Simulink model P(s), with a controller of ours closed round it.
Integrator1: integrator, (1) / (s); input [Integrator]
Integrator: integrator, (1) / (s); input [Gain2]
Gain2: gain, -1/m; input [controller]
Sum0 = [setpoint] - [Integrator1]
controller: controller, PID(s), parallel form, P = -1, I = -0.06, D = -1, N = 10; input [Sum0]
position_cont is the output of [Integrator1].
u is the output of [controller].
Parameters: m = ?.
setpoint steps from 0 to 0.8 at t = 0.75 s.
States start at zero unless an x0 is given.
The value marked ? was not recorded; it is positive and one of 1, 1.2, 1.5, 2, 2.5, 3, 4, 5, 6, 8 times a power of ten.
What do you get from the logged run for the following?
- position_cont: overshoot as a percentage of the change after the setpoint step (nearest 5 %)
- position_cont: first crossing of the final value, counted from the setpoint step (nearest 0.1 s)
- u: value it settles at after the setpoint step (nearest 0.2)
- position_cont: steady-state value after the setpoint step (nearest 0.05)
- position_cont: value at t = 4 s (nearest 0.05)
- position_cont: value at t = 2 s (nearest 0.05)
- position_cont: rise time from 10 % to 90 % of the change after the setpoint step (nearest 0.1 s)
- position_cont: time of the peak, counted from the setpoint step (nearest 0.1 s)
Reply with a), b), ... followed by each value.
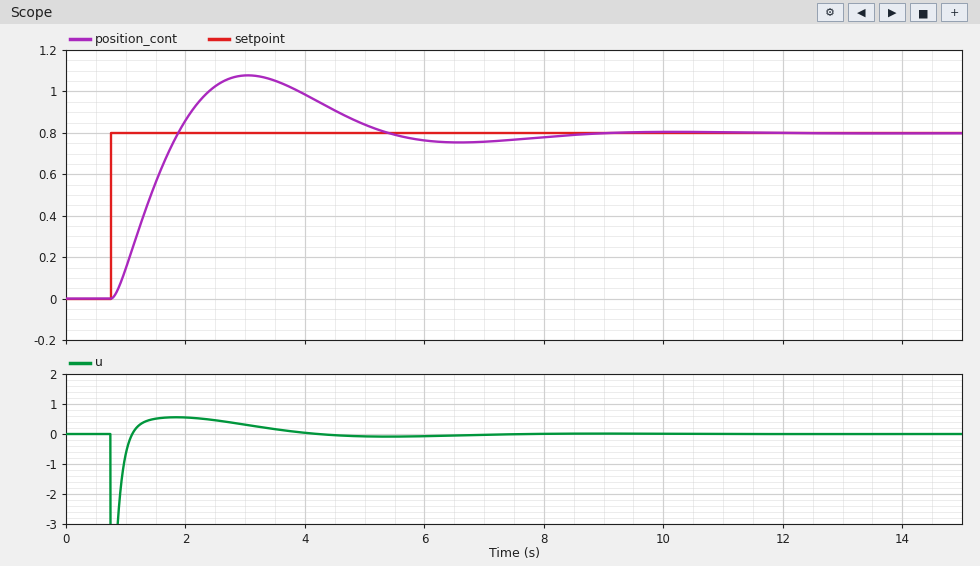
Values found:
a) 35 %
b) 1.1 s
c) 0.0
d) 0.80
e) 1.00
f) 0.85
g) 0.8 s
h) 2.3 s
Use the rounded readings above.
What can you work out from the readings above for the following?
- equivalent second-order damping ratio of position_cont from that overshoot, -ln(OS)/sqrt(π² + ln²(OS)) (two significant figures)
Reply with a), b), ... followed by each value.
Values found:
a) 0.32
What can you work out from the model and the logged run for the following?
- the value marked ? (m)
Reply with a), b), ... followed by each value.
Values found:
a) 1
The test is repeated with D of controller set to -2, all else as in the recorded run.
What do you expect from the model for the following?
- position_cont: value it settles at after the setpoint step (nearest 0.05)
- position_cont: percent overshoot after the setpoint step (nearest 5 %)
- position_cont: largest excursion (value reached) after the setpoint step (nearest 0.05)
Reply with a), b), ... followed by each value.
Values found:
a) 0.80
b) 15 %
c) 0.95
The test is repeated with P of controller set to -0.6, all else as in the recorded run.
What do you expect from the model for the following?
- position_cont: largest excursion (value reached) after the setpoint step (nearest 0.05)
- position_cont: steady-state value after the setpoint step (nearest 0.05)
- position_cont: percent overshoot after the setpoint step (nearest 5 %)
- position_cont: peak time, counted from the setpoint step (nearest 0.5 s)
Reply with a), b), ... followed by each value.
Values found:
a) 1.05
b) 0.80
c) 30 %
d) 3.0 s
